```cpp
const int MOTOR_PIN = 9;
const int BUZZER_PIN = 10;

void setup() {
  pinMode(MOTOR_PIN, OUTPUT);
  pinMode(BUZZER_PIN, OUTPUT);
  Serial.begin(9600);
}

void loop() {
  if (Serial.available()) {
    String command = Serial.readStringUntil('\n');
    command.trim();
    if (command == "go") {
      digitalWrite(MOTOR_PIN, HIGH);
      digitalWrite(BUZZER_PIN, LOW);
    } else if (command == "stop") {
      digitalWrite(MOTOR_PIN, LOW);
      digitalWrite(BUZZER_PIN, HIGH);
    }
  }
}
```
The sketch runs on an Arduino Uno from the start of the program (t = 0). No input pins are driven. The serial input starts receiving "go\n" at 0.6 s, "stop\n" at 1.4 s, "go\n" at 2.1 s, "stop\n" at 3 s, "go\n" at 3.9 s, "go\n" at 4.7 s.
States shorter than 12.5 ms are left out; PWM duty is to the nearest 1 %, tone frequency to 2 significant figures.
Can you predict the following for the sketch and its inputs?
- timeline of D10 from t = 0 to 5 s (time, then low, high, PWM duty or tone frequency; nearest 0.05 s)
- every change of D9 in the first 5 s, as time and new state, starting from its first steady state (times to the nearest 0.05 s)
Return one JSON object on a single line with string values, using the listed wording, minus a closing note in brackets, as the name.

{"timeline of D10 from t = 0 to 5 s": "0 s low; 1.4 s high; 2.1 s low; 3 s high; 3.9 s low", "every change of D9 in the first 5 s, as time and new state, starting from its first steady state": "0 s low; 0.6 s high; 1.4 s low; 2.1 s high; 3 s low; 3.9 s high"}
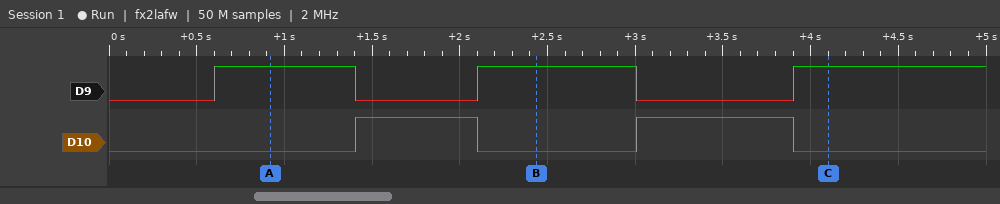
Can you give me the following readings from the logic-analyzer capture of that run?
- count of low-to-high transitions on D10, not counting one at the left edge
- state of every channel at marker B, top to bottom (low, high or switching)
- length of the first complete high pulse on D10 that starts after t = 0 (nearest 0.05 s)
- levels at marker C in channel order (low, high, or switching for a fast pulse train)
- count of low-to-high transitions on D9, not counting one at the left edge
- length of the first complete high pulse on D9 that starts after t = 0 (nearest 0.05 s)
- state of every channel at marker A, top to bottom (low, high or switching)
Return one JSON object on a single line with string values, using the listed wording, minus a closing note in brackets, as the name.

{"count of low-to-high transitions on D10, not counting one at the left edge": "2", "state of every channel at marker B, top to bottom": "D9 high, D10 low", "length of the first complete high pulse on D10 that starts after t = 0": "0.70 s", "levels at marker C in channel order": "D9 high, D10 low", "count of low-to-high transitions on D9, not counting one at the left edge": "3", "length of the first complete high pulse on D9 that starts after t = 0": "0.80 s", "state of every channel at marker A, top to bottom": "D9 high, D10 low"}
